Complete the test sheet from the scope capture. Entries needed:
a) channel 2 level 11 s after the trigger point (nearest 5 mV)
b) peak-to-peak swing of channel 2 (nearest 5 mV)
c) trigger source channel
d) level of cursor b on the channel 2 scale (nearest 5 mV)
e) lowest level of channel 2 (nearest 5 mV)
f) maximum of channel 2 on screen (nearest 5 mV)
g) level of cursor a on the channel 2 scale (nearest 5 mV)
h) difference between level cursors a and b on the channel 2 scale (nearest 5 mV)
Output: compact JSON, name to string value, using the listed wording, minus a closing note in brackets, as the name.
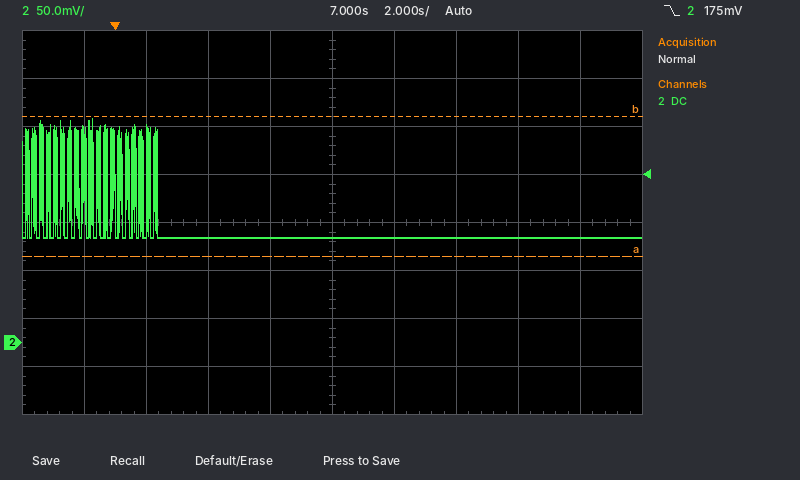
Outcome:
{"channel 2 level 11 s after the trigger point": "110 mV", "peak-to-peak swing of channel 2": "125 mV", "trigger source channel": "channel 2", "level of cursor b on the channel 2 scale": "235 mV", "lowest level of channel 2": "110 mV", "maximum of channel 2 on screen": "235 mV", "level of cursor a on the channel 2 scale": "90 mV", "difference between level cursors a and b on the channel 2 scale": "145 mV"}
